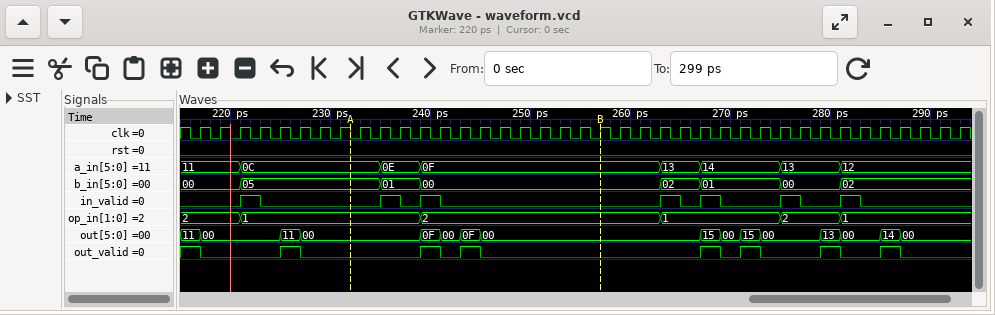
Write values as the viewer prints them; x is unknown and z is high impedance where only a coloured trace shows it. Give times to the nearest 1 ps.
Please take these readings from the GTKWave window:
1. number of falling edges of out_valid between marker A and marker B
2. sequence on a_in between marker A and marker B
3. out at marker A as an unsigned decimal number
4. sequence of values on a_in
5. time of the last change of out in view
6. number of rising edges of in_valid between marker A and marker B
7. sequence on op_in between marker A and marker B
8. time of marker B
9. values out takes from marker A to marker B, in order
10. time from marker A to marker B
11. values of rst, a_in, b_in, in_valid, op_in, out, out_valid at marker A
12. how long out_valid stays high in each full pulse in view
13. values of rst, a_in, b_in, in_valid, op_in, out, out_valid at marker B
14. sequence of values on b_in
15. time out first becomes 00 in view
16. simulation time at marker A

2
0C, 0E, 0F
0
11, 0C, 0E, 0F, 13, 14, 13, 12
287 ps
2
1, 2
257 ps
00, 0F, 00, 0F, 00
25 ps
rst=0, a_in=0C, b_in=05, in_valid=0, op_in=1, out=00, out_valid=0
2 ps, 2 ps, 2 ps, 2 ps, 2 ps, 2 ps, 2 ps
rst=0, a_in=0F, b_in=00, in_valid=0, op_in=2, out=00, out_valid=0
00, 05, 01, 00, 02, 01, 00, 02
217 ps
232 ps
